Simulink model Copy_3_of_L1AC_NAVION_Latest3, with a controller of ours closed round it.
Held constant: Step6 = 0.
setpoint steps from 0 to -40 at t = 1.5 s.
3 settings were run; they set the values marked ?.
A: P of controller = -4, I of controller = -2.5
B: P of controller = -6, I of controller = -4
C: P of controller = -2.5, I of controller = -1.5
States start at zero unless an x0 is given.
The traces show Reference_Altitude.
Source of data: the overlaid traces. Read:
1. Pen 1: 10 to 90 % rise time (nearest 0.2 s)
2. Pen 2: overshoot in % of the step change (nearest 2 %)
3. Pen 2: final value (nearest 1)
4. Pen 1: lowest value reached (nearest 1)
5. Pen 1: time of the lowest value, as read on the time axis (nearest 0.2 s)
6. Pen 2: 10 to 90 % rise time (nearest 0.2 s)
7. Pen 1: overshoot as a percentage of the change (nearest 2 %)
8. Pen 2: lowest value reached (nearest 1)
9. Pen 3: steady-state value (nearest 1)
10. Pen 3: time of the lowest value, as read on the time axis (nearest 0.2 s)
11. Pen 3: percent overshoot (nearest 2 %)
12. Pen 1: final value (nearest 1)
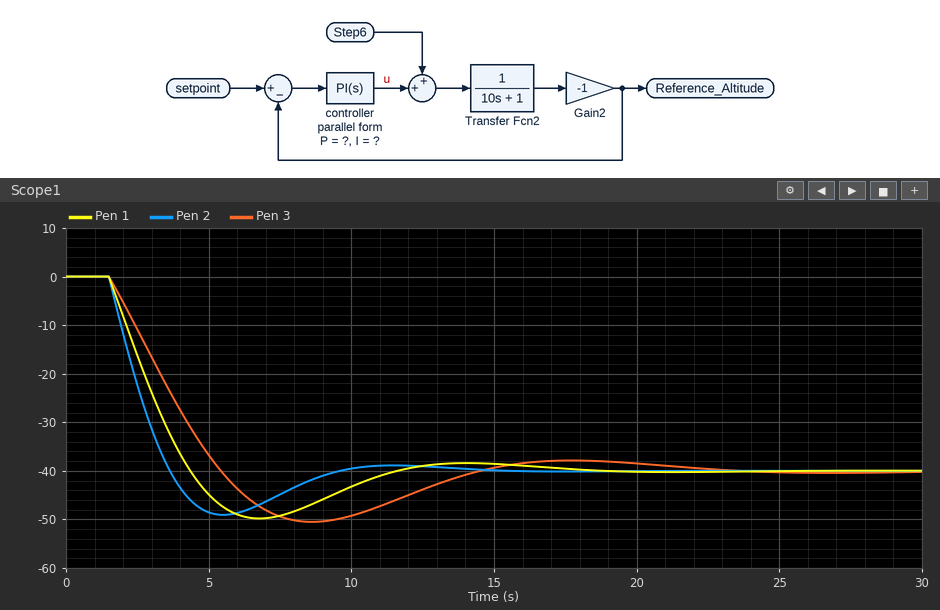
2.2 s
22 %
-40
-50
6.8 s
1.6 s
24 %
-49
-40
8.6 s
26 %
-40
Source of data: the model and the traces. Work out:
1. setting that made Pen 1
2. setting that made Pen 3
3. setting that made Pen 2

A
C
B
